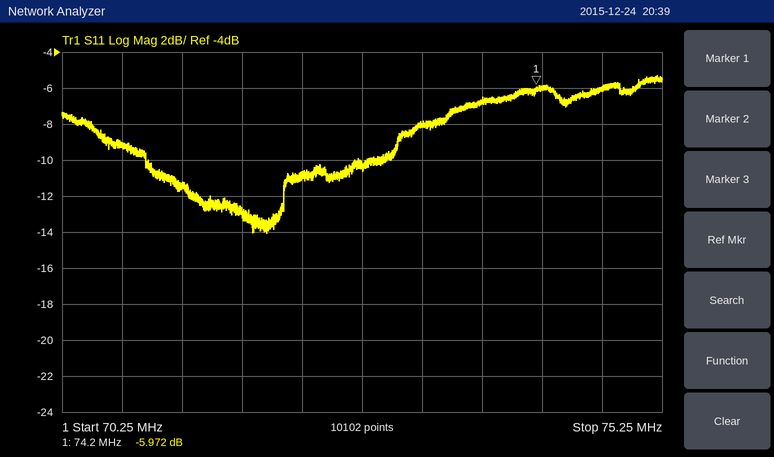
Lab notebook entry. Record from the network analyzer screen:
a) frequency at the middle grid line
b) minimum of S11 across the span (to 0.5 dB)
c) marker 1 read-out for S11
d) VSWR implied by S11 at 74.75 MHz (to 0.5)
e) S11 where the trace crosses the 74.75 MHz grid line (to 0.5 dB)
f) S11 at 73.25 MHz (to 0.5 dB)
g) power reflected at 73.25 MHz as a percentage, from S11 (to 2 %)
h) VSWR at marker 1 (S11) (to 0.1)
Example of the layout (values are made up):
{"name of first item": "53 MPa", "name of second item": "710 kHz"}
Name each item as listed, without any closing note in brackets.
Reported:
{"frequency at the middle grid line": "72.75 MHz", "minimum of S11 across the span": "-14.0 dB", "marker 1 read-out for S11": "-5.972 dB", "VSWR implied by S11 at 74.75 MHz": "3.0", "S11 where the trace crosses the 74.75 MHz grid line": "-6.0 dB", "S11 at 73.25 MHz": "-8.0 dB", "power reflected at 73.25 MHz as a percentage, from S11": "16 %", "VSWR at marker 1 (S11)": "3.0"}
